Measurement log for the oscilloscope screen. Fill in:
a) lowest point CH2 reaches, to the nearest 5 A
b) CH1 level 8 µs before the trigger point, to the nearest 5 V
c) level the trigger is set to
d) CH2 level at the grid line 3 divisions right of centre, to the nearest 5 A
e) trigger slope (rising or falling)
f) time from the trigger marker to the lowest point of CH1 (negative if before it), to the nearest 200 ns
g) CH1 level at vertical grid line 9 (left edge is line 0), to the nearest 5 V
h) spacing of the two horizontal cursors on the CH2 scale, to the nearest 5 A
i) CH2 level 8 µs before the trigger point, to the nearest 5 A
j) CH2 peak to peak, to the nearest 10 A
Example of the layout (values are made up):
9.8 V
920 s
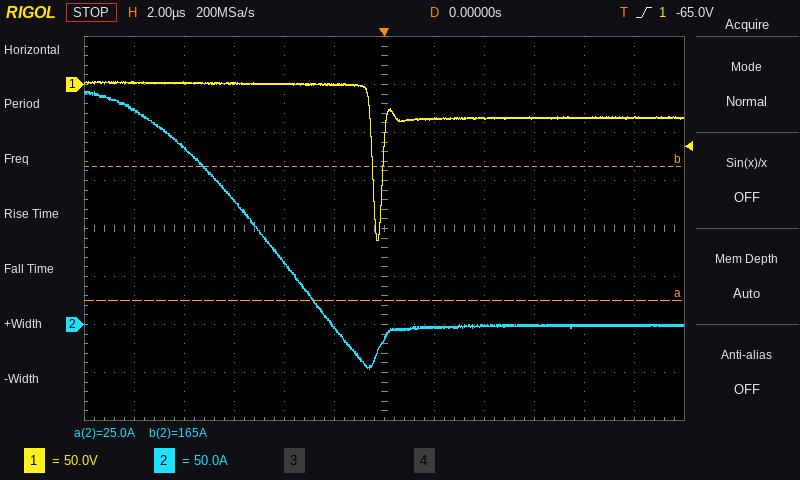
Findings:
-45 A
0 V
-65.0 V
0 A
rising
-200 ns
-35 V
140 A
185 A
290 A
